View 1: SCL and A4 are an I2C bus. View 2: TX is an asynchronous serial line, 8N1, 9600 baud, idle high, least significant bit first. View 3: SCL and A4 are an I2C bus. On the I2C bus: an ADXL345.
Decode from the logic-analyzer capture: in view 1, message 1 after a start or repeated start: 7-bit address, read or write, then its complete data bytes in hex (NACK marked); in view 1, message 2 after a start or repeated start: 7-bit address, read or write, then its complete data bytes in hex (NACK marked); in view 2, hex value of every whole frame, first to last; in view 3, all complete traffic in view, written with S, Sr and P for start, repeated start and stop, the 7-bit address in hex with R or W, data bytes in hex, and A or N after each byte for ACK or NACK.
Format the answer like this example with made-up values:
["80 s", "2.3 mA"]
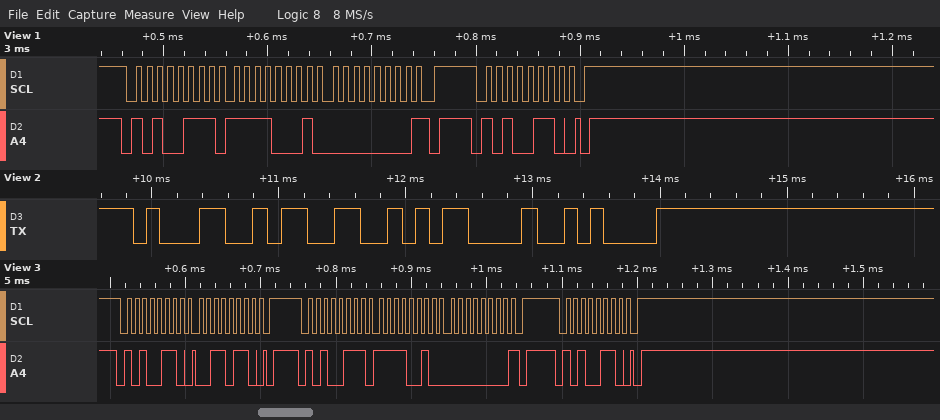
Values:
["0x53 read: F1 00 NACK", "0x53 write", "31 33 0D 0A", "S 53W A 36 A P S 53R A F2 A 00 N P S 53W A P"]
